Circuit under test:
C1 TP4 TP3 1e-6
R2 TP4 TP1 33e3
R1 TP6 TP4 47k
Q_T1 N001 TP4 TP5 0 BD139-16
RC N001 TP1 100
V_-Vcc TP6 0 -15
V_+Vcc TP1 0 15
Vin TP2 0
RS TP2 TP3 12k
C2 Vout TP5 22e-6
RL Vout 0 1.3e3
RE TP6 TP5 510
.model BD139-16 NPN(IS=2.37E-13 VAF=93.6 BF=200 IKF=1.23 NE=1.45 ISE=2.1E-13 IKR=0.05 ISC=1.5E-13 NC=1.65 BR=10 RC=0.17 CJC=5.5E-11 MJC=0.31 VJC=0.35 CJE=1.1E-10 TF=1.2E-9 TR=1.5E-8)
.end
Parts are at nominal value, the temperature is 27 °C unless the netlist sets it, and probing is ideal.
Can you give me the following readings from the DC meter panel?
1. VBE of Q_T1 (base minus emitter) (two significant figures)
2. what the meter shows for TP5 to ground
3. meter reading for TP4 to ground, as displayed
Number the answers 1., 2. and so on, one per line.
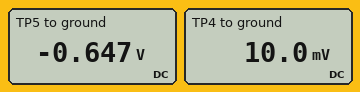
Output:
1. 660 mV
2. -0.647 V
3. 10.0 mV
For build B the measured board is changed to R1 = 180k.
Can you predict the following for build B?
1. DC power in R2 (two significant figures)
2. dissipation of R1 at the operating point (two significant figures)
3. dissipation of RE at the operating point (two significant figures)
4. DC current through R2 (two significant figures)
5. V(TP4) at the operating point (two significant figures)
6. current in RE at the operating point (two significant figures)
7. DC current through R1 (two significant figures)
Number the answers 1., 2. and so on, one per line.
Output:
1. 3.0 mW
2. 2.2 mW
3. 730 mW
4. 300 µA
5. 5.0 V
6. 38 mA
7. 110 µA
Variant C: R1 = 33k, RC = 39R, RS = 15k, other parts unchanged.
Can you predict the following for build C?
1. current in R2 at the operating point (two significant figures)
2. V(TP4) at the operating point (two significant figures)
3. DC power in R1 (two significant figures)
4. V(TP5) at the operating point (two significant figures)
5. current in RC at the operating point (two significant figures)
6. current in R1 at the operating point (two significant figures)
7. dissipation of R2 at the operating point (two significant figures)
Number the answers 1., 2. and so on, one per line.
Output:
1. 510 µA
2. -1.9 V
3. 5.2 mW
4. -2.5 V
5. 24 mA
6. 400 µA
7. 8.6 mW
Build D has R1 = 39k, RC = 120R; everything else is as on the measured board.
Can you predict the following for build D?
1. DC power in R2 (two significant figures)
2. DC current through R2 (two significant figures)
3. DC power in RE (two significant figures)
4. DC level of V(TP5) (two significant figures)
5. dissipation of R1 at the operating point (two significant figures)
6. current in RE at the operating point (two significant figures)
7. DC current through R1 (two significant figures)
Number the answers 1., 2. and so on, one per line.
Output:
1. 7.7 mW
2. 480 µA
3. 350 mW
4. -1.6 V
5. 5.0 mW
6. 26 mA
7. 360 µA
